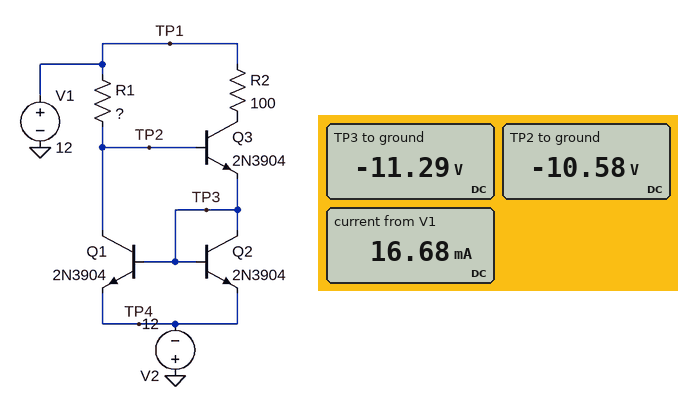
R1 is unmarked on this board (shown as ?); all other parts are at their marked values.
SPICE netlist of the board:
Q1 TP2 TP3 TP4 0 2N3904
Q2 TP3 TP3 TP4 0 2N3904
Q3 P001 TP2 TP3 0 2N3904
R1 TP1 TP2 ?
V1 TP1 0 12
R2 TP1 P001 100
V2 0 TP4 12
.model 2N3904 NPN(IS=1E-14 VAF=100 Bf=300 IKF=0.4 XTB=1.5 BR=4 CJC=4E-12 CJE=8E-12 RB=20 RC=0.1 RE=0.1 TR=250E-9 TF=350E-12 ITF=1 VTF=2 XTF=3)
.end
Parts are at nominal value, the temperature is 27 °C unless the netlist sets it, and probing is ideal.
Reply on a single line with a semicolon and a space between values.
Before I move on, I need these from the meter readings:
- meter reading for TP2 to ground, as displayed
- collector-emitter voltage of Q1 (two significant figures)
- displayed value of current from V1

-10.58 V; 1.4 V; 16.68 mA
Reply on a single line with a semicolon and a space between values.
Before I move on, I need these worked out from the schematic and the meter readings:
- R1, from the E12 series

2.7 kΩ
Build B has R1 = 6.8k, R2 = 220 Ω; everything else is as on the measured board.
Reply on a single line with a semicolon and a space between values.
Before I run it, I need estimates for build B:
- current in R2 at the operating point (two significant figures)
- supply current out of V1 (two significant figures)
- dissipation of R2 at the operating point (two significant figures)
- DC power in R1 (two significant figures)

3.3 mA; 6.6 mA; 2.4 mW; 75 mW
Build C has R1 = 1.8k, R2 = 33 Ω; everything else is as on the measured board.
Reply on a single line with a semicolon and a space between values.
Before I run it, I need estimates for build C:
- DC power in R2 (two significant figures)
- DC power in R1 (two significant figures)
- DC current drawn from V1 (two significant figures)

5.1 mW; 280 mW; 25 mA
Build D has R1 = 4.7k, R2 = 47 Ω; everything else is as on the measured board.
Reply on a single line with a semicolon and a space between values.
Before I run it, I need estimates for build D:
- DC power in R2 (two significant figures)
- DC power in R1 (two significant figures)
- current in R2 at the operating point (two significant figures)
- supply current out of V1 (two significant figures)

1.1 mW; 110 mW; 4.8 mA; 9.6 mA
